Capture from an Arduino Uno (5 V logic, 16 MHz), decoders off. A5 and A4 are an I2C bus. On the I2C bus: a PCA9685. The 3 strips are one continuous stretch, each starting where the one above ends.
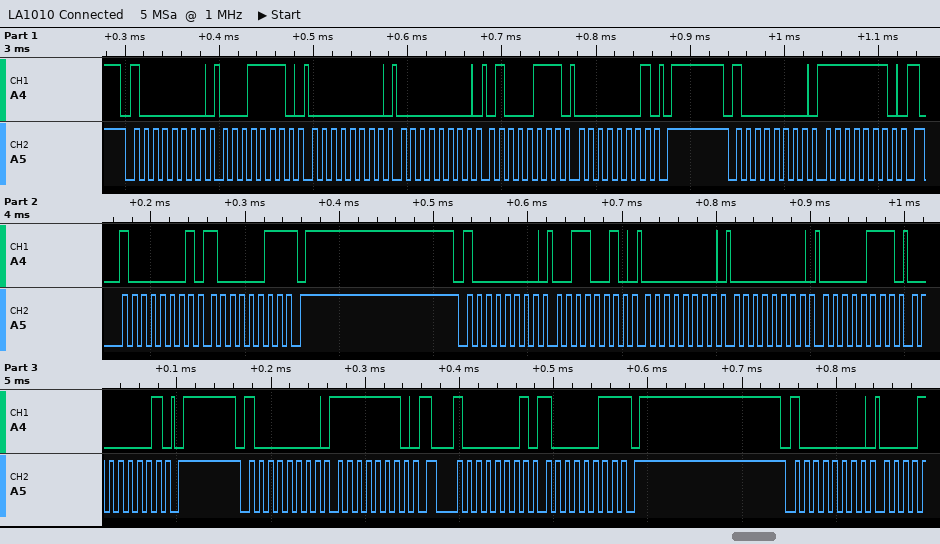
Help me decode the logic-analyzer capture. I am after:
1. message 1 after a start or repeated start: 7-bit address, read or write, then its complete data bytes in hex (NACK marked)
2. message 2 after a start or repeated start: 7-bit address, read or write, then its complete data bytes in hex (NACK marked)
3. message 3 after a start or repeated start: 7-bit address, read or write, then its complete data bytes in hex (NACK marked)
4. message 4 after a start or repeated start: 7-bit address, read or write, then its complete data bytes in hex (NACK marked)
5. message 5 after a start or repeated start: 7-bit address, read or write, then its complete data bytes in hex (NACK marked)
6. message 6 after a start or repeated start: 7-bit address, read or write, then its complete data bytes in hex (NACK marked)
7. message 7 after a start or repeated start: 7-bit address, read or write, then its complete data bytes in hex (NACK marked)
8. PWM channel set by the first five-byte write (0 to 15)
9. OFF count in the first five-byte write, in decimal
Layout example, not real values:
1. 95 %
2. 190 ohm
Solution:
1. 0x40 write: 1E 00 00 47 01
2. 0x40 write: FE
3. 0x40 read: 83 NACK
4. 0x40 write: 32 00 00 07 01
5. 0x40 write: FE
6. 0x40 read: 83 NACK
7. 0x40 write
8. 6
9. 327
